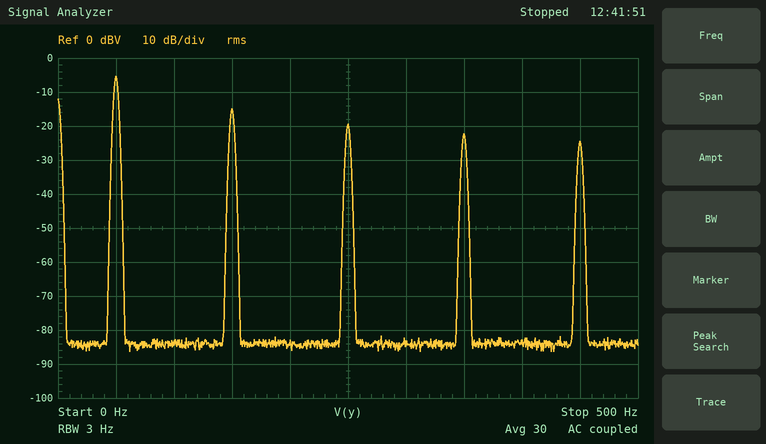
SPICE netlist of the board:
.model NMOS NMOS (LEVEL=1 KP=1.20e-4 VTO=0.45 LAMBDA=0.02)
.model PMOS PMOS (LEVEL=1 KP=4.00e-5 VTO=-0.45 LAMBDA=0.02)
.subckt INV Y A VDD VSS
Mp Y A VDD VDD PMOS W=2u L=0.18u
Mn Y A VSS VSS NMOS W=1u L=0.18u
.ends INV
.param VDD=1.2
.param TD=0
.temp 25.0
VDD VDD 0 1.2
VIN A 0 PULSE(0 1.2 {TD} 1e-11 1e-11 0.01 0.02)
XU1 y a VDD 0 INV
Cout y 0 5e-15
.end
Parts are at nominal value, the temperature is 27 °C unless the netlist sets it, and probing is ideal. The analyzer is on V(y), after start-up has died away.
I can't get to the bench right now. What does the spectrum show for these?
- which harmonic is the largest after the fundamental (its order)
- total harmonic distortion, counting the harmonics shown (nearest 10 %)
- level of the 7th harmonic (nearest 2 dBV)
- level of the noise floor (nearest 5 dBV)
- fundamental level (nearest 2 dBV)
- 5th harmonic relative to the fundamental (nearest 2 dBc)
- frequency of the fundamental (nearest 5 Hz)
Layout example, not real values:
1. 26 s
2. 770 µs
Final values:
1. 3
2. 40 %
3. -22 dBV
4. -85 dBV
5. -6 dBV
6. -14 dBc
7. 50 Hz
